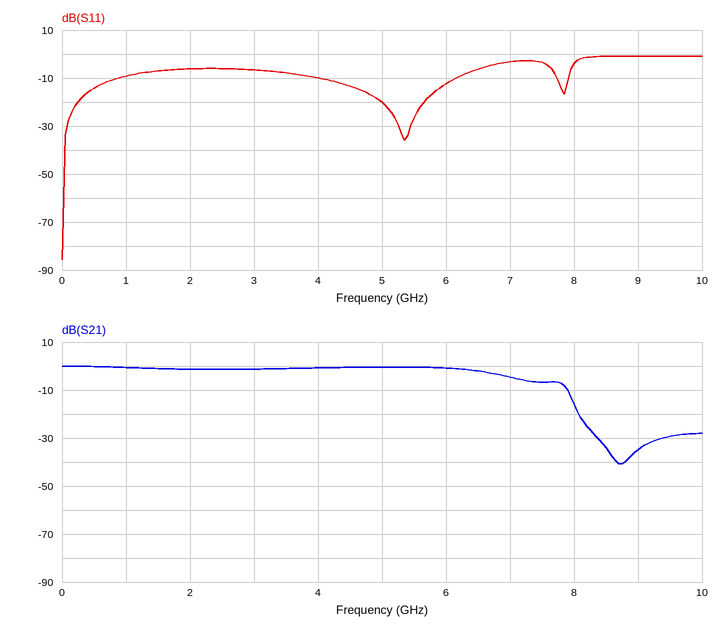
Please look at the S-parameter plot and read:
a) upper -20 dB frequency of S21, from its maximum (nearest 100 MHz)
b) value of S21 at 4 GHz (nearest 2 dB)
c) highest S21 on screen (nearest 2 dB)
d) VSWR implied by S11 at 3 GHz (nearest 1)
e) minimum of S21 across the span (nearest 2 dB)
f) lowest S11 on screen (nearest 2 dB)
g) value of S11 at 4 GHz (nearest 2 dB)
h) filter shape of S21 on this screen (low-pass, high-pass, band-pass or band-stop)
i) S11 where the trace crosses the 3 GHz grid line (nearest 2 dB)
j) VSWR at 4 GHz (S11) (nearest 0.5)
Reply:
8.1 GHz
0 dB
0 dB
3
-40 dB
-86 dB
-10 dB
low-pass
-6 dB
2.0
